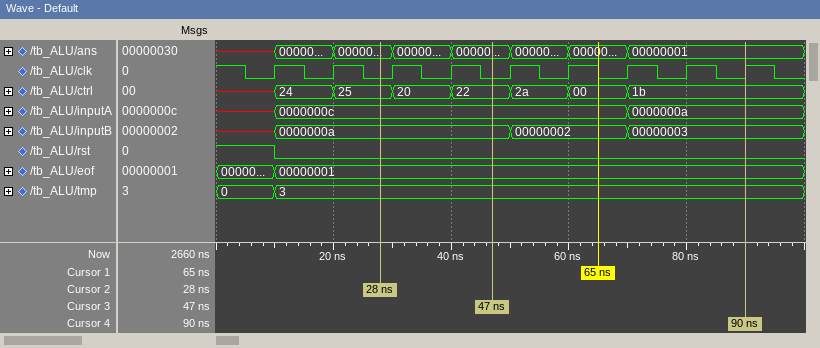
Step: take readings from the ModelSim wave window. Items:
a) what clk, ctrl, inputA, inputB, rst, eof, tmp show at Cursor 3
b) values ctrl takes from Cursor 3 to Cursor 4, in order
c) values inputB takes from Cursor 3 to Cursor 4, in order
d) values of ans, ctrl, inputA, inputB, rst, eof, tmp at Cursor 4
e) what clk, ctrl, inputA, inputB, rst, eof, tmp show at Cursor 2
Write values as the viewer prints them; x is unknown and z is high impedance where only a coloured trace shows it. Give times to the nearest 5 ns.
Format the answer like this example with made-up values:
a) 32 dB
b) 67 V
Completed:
a) clk=0, ctrl=22, inputA=0000000c, inputB=0000000a, rst=0, eof=00000001, tmp=3
b) 22, 2a, 00, 1b
c) 0000000a, 00000002, 00000003
d) ans=00000001, ctrl=1b, inputA=0000000a, inputB=00000003, rst=0, eof=00000001, tmp=3
e) clk=0, ctrl=25, inputA=0000000c, inputB=0000000a, rst=0, eof=00000001, tmp=3
